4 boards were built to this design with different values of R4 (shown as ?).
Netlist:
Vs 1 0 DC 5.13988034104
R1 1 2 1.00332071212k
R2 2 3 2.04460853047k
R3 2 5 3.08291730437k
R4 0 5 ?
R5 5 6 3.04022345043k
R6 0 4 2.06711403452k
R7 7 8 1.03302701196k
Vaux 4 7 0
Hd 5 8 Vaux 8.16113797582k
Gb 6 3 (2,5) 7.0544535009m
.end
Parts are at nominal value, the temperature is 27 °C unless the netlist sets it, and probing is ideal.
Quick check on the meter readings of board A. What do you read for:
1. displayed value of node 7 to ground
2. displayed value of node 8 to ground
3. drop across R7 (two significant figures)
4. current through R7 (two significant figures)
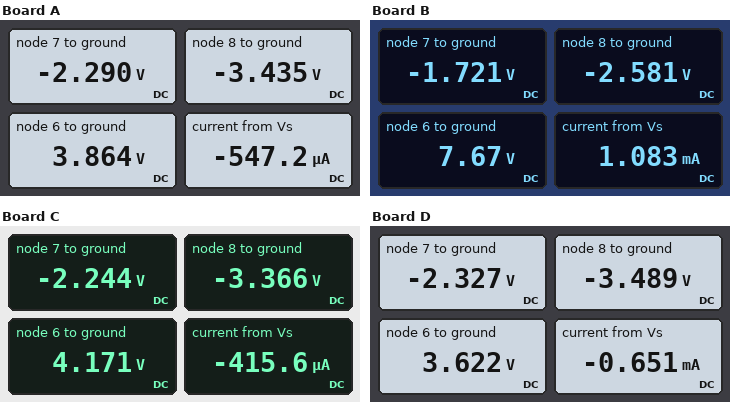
-2.290 V
-3.435 V
1.1 V
1.1 mA
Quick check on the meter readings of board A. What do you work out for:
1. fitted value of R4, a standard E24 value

10 kΩ
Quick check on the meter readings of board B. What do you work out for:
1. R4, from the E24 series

2.2 kΩ
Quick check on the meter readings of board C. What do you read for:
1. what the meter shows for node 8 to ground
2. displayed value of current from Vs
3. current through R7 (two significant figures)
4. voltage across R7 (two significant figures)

-3.366 V
-415.6 µA
1.1 mA
1.1 V
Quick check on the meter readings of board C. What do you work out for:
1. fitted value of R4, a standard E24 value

8.2 kΩ
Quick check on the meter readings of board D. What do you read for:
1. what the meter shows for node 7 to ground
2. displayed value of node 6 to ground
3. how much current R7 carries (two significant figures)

-2.327 V
3.622 V
1.1 mA
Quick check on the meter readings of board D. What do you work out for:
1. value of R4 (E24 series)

12 kΩ
